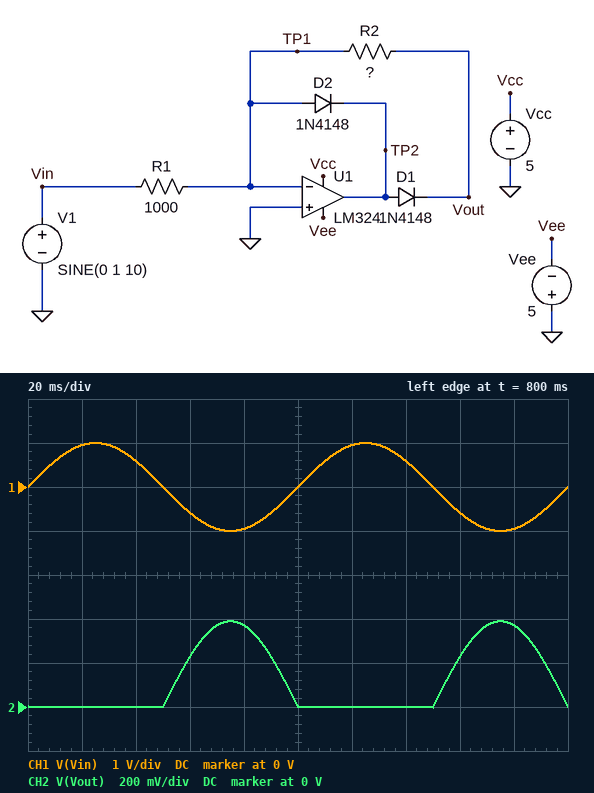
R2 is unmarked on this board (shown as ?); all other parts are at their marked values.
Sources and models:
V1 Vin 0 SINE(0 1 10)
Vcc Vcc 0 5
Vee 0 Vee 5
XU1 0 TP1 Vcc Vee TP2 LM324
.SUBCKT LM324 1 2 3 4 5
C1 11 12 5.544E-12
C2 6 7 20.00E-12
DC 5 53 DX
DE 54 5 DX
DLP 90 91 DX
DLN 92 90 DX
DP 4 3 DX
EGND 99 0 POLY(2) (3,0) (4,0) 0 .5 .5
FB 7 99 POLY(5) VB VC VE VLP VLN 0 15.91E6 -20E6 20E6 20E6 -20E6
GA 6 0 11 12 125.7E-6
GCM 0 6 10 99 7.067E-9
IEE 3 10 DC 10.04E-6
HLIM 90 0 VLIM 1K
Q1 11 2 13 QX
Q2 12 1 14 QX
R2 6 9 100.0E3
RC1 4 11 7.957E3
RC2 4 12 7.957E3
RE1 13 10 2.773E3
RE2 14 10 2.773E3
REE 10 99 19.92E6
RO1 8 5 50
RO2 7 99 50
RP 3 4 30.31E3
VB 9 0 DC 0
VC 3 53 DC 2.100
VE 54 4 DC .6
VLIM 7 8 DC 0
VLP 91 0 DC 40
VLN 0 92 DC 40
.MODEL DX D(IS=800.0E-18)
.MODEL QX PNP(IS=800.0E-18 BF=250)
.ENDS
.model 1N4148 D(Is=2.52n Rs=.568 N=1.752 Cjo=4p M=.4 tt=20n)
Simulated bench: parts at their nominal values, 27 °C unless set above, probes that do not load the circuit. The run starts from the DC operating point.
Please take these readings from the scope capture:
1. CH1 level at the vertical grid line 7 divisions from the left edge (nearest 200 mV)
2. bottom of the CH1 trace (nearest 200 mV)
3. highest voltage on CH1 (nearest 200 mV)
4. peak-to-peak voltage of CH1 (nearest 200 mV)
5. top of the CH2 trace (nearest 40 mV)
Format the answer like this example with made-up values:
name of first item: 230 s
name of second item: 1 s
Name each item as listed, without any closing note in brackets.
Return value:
CH1 level at the vertical grid line 7 divisions from the left edge: 600 mV
bottom of the CH1 trace: -1.0 V
highest voltage on CH1: 1.0 V
peak-to-peak voltage of CH1: 2.0 V
top of the CH2 trace: 400 mV
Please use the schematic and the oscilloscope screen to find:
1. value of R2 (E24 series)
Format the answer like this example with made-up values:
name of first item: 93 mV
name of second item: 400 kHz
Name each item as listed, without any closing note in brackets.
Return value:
value of R2: 390 Ω
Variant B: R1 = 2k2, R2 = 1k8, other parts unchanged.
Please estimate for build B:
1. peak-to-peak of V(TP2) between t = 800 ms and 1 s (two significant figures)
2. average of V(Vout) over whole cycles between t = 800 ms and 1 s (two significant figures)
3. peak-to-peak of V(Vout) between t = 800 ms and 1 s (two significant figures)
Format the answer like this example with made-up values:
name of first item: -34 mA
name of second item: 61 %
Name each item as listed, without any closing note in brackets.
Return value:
peak-to-peak of V(TP2) between t = 800 ms and 1 s: 1.9 V
average of V(Vout) over whole cycles between t = 800 ms and 1 s: 260 mV
peak-to-peak of V(Vout) between t = 800 ms and 1 s: 820 mV
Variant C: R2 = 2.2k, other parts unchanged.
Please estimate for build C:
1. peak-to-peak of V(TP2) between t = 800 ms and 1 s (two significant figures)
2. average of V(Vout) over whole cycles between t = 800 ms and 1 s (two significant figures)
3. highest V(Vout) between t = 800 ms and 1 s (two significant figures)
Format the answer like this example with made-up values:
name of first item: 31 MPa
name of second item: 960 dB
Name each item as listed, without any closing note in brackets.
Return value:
peak-to-peak of V(TP2) between t = 800 ms and 1 s: 3.4 V
average of V(Vout) over whole cycles between t = 800 ms and 1 s: 700 mV
highest V(Vout) between t = 800 ms and 1 s: 2.2 V
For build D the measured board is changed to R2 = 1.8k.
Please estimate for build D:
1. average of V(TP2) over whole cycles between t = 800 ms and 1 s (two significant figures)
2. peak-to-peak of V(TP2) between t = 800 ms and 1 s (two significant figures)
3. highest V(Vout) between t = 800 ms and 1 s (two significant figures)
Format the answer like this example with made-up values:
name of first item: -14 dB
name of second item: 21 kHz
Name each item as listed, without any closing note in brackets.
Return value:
average of V(TP2) over whole cycles between t = 800 ms and 1 s: 570 mV
peak-to-peak of V(TP2) between t = 800 ms and 1 s: 3.0 V
highest V(Vout) between t = 800 ms and 1 s: 1.8 V
